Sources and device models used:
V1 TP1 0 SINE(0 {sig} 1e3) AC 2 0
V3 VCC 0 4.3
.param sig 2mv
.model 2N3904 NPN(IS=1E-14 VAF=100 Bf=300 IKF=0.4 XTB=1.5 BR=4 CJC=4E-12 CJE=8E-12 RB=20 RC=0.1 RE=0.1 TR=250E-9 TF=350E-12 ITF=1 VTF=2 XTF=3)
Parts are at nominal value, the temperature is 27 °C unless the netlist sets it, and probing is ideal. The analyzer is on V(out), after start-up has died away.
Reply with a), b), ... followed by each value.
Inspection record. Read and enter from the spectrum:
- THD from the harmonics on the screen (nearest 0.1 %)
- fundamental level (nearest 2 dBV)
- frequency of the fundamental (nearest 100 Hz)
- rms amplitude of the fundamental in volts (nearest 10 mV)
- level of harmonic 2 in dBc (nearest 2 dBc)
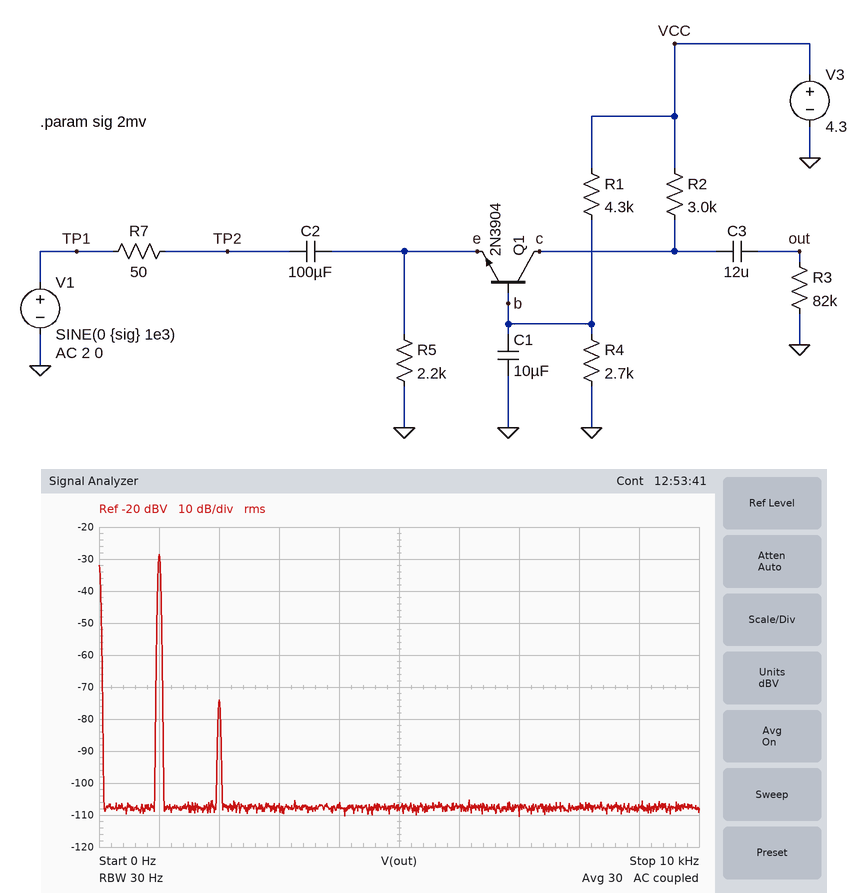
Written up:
a) 0.5 %
b) -28 dBV
c) 1.0 kHz
d) 40 mV
e) -46 dBc
